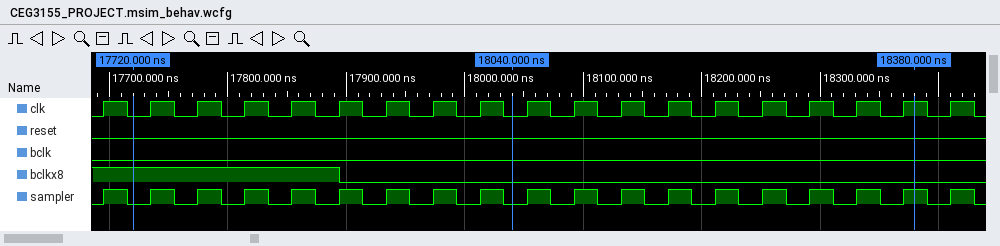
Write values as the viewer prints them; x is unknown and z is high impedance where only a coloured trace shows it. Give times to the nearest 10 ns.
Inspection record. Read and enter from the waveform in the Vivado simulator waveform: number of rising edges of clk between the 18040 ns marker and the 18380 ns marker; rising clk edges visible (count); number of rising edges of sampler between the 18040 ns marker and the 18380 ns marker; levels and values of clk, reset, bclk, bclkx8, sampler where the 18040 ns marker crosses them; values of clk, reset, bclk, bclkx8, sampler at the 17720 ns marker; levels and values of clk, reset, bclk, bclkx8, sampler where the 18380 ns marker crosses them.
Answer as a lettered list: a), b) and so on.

a) 9
b) 19
c) 9
d) clk=0, reset=0, bclk=0, bclkx8=0, sampler=0
e) clk=0, reset=0, bclk=0, bclkx8=1, sampler=0
f) clk=1, reset=0, bclk=0, bclkx8=0, sampler=1
